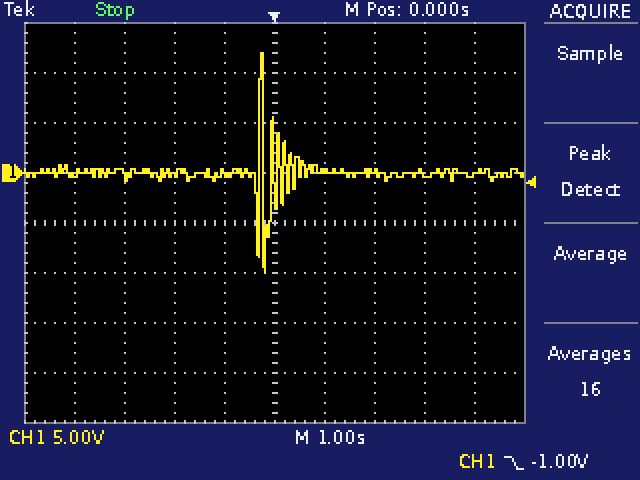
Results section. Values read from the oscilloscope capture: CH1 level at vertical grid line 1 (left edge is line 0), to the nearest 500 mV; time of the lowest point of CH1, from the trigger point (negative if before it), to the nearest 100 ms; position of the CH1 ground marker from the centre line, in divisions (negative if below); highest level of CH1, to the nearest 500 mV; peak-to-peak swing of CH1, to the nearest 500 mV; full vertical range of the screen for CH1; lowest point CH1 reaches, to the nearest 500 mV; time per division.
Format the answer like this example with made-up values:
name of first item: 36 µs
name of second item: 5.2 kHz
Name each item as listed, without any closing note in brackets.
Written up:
CH1 level at vertical grid line 1 (left edge is line 0), to the nearest 500 mV: 0.0 V
time of the lowest point of CH1, from the trigger point (negative if before it), to the nearest 100 ms: -200 ms
position of the CH1 ground marker from the centre line, in divisions: +1.0 div
highest level of CH1, to the nearest 500 mV: 12.0 V
peak-to-peak swing of CH1, to the nearest 500 mV: 22.0 V
full vertical range of the screen for CH1: 40 V
lowest point CH1 reaches, to the nearest 500 mV: -10.0 V
time per division: 1 s
